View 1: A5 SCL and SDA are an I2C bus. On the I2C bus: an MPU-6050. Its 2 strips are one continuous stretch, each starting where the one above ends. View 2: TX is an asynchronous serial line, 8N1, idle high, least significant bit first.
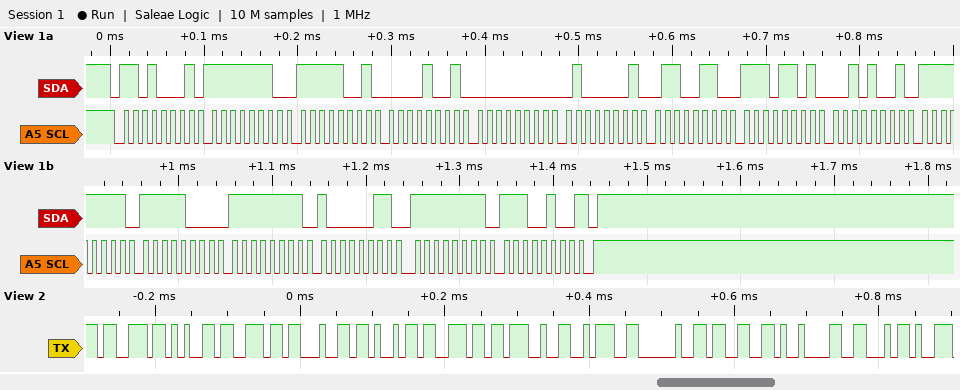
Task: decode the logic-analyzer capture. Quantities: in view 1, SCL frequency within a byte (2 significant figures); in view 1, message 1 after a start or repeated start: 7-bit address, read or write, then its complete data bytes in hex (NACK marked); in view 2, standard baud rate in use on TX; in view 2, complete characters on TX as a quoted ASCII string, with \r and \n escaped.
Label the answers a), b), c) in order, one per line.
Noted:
a) 100 kHz
b) 0x68 read: FE F9 09 00 41 66 ED 29 FF F8 FF 83 FF E4 NACK
c) 115200 baud
d) "sendin': 3\tF"
